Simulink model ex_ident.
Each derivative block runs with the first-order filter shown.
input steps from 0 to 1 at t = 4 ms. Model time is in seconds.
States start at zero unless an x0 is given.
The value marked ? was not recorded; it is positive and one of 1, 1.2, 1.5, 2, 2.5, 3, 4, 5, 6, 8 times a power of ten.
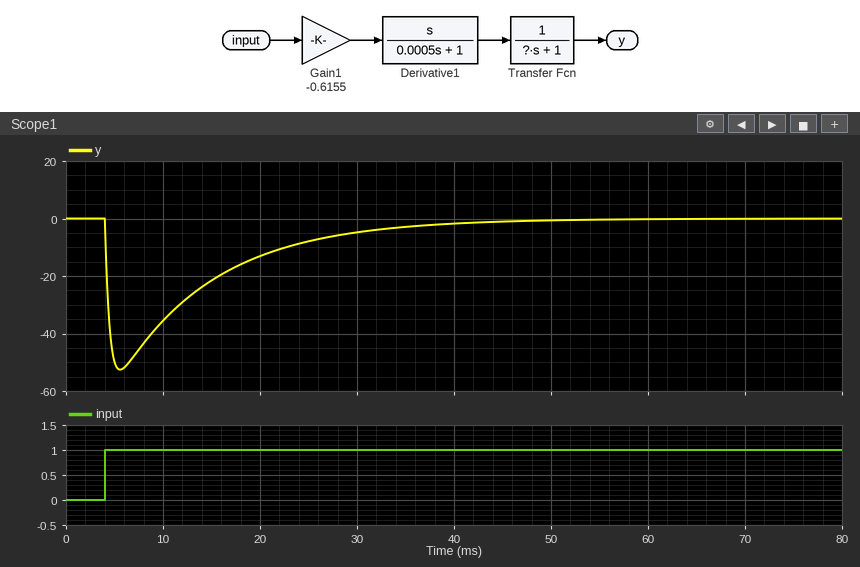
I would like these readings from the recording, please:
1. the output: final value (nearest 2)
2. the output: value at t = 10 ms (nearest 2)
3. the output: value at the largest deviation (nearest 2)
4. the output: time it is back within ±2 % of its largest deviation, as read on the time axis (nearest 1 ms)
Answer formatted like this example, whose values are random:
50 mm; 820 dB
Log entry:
0; -36; -52; 45 ms
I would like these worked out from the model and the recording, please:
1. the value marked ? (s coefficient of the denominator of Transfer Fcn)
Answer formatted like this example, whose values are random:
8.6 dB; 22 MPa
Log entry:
0.01
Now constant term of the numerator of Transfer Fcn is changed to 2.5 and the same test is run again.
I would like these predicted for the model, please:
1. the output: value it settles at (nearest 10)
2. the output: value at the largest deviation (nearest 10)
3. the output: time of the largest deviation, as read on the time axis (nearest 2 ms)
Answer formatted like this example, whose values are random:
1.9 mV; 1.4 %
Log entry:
0; -130; 6 ms
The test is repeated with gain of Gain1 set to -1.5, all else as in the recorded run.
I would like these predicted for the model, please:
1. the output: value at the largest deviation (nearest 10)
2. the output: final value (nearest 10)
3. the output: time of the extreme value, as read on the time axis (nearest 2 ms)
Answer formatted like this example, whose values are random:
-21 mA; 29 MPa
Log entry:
-130; 0; 6 ms
